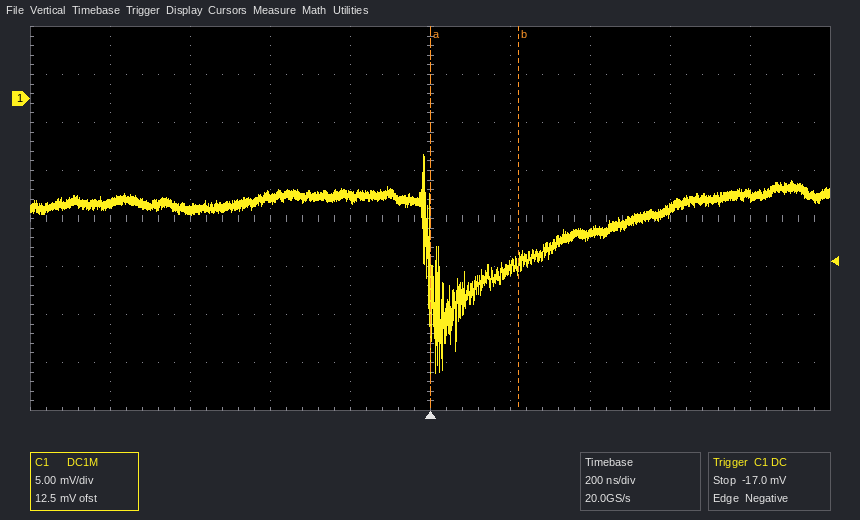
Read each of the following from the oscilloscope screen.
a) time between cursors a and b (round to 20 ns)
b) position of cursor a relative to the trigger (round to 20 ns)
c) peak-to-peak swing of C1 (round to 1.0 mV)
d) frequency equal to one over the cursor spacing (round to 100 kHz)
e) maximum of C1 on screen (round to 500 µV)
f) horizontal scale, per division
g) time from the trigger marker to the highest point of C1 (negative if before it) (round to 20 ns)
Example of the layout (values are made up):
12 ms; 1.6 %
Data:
220 ns; 0 ns; 23.0 mV; 4.5 MHz; -6.0 mV; 200 ns; -20 ns
